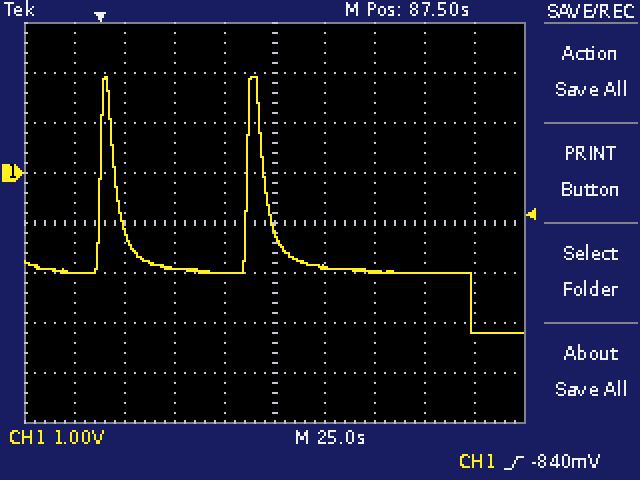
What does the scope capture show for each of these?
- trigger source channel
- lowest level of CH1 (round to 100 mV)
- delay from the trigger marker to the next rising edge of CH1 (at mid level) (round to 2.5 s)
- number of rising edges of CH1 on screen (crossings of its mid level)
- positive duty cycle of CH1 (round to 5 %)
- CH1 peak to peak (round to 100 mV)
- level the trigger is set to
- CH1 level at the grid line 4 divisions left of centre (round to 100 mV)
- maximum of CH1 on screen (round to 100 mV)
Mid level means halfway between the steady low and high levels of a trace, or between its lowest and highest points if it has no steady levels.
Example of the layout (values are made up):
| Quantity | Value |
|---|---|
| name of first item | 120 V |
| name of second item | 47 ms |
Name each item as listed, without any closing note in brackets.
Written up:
| Quantity | Value |
|---|---|
| trigger source channel | CH1 |
| lowest level of CH1 | -3.2 V |
| delay from the trigger marker to the next rising edge of CH1 (at mid level) | 72.5 s |
| number of rising edges of CH1 on screen | 2 |
| positive duty cycle of CH1 | 15 % |
| CH1 peak to peak | 5.1 V |
| level the trigger is set to | -840 mV |
| CH1 level at the grid line 4 divisions left of centre | -2.0 V |
| maximum of CH1 on screen | 1.9 V |
